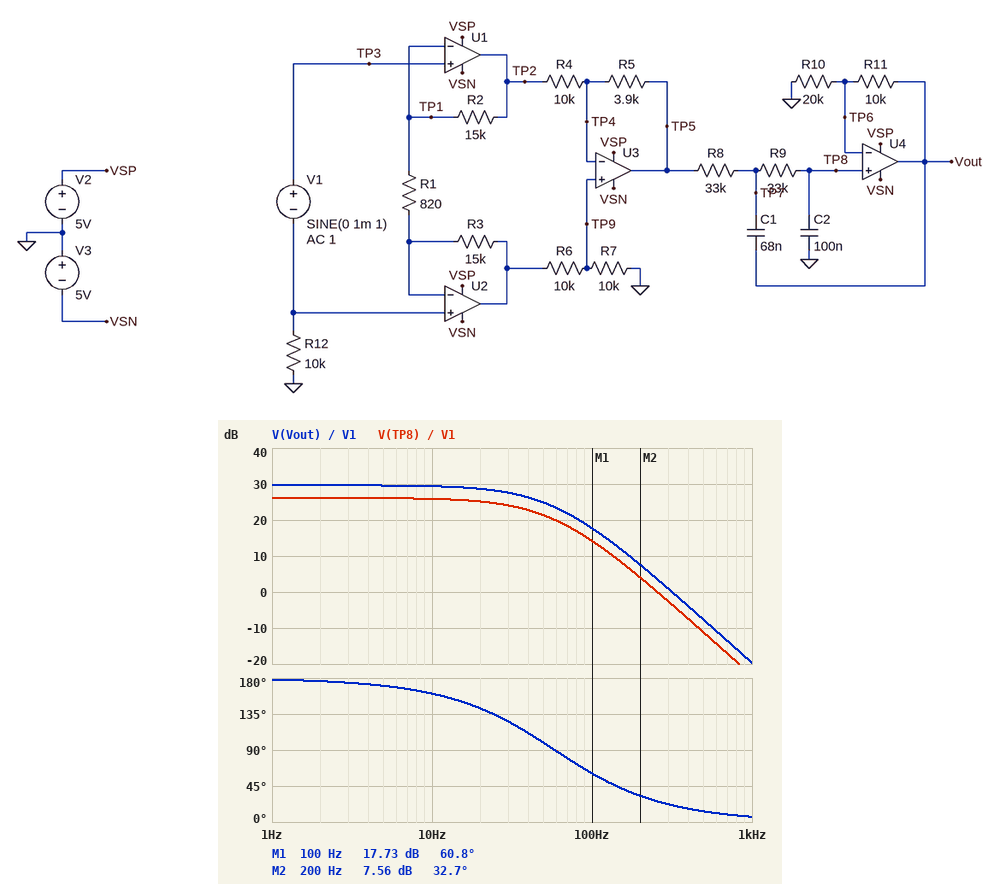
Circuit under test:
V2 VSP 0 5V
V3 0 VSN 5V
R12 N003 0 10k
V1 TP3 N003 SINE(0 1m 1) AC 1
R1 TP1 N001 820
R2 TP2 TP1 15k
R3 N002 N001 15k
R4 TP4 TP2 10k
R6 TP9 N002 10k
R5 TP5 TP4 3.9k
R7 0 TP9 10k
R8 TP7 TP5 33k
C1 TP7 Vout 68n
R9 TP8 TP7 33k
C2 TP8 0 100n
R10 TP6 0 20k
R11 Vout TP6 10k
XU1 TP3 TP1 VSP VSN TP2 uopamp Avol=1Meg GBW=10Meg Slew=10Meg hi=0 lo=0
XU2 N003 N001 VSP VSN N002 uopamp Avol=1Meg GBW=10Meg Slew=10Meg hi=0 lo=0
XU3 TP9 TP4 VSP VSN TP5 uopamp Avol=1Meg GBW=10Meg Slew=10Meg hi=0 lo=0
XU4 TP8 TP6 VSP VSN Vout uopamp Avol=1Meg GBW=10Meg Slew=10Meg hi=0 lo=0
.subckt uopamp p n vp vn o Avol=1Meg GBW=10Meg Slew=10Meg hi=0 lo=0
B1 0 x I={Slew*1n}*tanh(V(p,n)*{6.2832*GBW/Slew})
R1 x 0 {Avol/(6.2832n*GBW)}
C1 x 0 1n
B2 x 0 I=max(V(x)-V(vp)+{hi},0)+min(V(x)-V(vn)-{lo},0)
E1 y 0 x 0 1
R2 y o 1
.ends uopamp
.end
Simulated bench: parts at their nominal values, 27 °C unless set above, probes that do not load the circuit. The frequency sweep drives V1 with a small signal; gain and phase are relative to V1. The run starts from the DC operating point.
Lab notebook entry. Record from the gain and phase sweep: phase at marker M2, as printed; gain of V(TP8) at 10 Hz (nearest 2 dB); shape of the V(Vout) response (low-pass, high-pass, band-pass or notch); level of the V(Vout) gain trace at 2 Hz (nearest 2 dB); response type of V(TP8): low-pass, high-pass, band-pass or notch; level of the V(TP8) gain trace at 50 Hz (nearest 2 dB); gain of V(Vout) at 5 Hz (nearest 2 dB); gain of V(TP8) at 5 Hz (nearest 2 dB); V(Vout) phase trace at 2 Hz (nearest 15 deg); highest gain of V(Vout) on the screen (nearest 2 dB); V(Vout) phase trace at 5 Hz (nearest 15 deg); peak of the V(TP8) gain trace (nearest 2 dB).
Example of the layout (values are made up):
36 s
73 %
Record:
32.7 deg
26 dB
low-pass
30 dB
low-pass
22 dB
30 dB
26 dB
180 deg
30 dB
165 deg
26 dB
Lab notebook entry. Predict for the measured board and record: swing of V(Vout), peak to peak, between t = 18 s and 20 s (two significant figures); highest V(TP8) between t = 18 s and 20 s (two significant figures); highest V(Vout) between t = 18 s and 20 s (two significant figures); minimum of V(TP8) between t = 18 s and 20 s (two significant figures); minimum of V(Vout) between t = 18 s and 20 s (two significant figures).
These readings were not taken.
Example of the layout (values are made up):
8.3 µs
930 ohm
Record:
61 mV
20 mV
30 mV
-20 mV
-30 mV
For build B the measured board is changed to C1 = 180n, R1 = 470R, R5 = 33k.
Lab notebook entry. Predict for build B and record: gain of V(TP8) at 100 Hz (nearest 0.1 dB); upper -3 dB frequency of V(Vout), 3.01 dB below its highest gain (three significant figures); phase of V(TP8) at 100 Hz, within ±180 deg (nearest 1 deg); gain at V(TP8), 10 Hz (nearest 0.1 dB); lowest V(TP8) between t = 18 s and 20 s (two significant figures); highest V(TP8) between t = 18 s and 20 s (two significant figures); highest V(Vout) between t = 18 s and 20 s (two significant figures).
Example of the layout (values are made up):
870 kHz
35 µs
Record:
27.9 dB
42.7 Hz
19 deg
45.4 dB
-180 mV
180 mV
270 mV
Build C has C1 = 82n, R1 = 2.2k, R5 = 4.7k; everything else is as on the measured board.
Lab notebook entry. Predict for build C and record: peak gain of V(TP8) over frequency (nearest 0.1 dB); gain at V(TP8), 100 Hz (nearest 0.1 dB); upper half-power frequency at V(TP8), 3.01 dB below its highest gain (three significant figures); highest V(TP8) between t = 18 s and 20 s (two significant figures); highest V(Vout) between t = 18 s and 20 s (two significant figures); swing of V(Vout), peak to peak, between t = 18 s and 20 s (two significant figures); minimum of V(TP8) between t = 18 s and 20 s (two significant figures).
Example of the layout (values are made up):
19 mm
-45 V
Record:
18.8 dB
6.4 dB
41.1 Hz
8.7 mV
13 mV
26 mV
-8.7 mV
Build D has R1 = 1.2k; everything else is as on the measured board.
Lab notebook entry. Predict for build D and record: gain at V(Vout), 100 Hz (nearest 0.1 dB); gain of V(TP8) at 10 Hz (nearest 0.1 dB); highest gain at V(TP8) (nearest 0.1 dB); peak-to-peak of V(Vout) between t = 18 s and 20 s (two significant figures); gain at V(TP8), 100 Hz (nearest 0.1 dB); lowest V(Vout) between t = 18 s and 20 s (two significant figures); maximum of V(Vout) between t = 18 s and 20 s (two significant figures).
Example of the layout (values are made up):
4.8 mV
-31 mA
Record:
14.5 dB
22.6 dB
22.9 dB
42 mV
11.0 dB
-21 mV
21 mV
